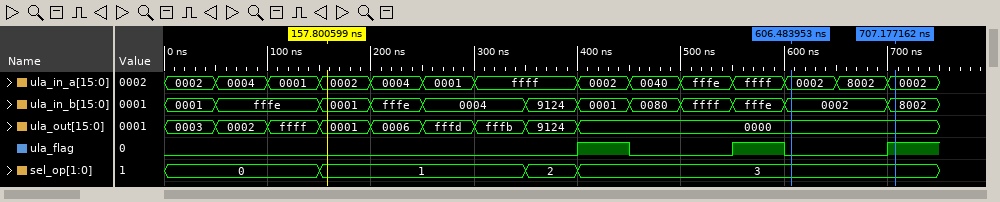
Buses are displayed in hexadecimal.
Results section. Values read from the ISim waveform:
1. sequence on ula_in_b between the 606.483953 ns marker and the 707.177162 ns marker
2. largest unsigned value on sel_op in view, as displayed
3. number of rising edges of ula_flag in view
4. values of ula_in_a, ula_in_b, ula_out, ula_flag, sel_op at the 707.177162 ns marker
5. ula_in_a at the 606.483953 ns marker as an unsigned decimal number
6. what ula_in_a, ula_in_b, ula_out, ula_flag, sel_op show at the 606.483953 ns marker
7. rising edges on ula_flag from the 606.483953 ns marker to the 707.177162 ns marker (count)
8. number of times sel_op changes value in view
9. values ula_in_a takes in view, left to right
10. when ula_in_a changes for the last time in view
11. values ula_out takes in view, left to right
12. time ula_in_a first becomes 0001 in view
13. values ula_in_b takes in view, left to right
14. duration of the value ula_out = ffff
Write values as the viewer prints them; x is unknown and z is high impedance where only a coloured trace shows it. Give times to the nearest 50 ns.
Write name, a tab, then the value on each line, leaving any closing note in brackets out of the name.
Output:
sequence on ula_in_b between the 606.483953 ns marker and the 707.177162 ns marker	0002, 8002
largest unsigned value on sel_op in view, as displayed	3
number of rising edges of ula_flag in view	3
values of ula_in_a, ula_in_b, ula_out, ula_flag, sel_op at the 707.177162 ns marker	ula_in_a=0002, ula_in_b=8002, ula_out=0000, ula_flag=1, sel_op=3
ula_in_a at the 606.483953 ns marker as an unsigned decimal number	2
what ula_in_a, ula_in_b, ula_out, ula_flag, sel_op show at the 606.483953 ns marker	ula_in_a=0002, ula_in_b=0002, ula_out=0000, ula_flag=0, sel_op=3
rising edges on ula_flag from the 606.483953 ns marker to the 707.177162 ns marker	1
number of times sel_op changes value in view	3
values ula_in_a takes in view, left to right	0002, 0004, 0001, 0002, 0004, 0001, ffff, 0002, 0040, fffe, ffff, 0002, 8002, 0002
when ula_in_a changes for the last time in view	700 ns
values ula_out takes in view, left to right	0003, 0002, ffff, 0001, 0006, fffd, fffb, 9124, 0000
time ula_in_a first becomes 0001 in view	100 ns
values ula_in_b takes in view, left to right	0001, fffe, 0001, fffe, 0004, 9124, 0001, 0080, ffff, fffe, 0002, 8002
duration of the value ula_out = ffff	50 ns
